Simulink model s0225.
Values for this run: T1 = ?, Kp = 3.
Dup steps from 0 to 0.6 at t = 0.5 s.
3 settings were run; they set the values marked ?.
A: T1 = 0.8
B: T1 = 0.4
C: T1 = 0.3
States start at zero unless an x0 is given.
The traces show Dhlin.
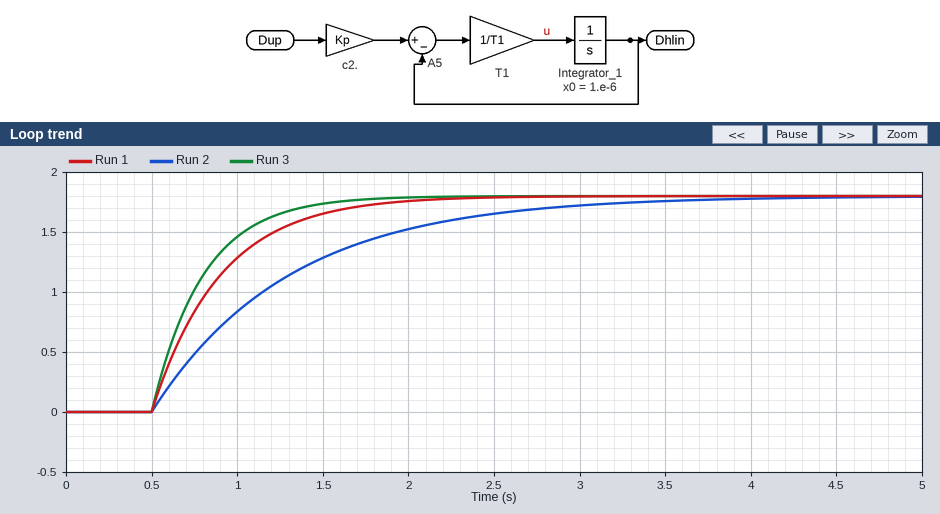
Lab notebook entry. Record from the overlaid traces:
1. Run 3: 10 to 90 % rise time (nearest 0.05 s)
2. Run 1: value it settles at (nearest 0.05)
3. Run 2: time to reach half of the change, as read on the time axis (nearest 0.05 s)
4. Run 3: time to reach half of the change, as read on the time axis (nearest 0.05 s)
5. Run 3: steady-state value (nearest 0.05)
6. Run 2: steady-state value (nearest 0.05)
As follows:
0.65 s
1.80
1.05 s
0.70 s
1.80
1.80
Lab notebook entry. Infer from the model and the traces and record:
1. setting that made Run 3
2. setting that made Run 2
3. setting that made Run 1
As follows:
C
A
B
